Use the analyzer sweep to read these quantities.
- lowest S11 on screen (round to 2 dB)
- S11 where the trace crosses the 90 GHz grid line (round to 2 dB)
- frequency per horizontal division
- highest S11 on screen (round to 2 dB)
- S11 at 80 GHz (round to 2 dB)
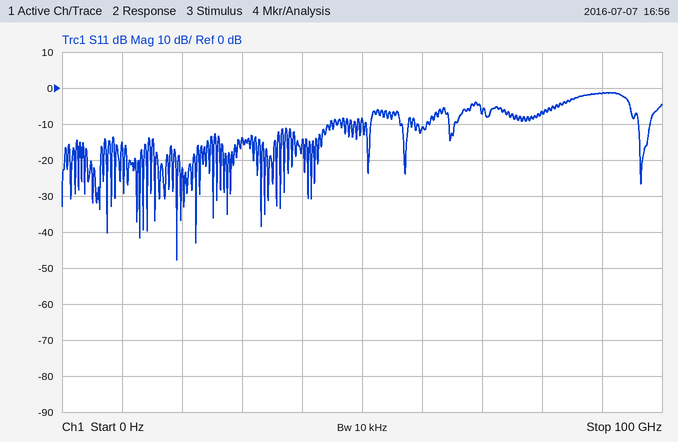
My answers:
-48 dB
-2 dB
10 GHz
-2 dB
-6 dB
